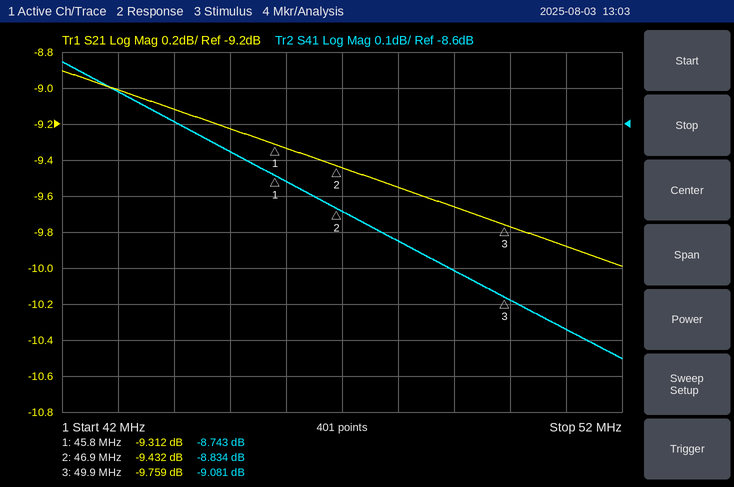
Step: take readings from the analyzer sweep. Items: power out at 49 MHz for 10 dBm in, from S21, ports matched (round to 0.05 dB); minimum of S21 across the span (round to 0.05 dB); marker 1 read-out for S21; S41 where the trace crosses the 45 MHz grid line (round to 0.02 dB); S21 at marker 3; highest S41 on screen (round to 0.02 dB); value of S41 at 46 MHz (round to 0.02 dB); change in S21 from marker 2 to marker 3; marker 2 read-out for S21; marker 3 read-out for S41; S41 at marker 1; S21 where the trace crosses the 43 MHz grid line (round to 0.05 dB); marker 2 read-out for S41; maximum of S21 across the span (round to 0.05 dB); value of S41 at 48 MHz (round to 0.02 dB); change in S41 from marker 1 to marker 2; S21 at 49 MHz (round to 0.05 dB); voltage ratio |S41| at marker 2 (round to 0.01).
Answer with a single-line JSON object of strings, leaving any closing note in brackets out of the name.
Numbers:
{"power out at 49 MHz for 10 dBm in, from S21, ports matched": "0.35 dBm", "minimum of S21 across the span": "-10.00 dB", "marker 1 read-out for S21": "-9.312 dB", "S41 where the trace crosses the 45 MHz grid line": "-8.68 dB", "S21 at marker 3": "-9.759 dB", "highest S41 on screen": "-8.42 dB", "value of S41 at 46 MHz": "-8.76 dB", "change in S21 from marker 2 to marker 3": "-0.327 dB", "marker 2 read-out for S21": "-9.432 dB", "marker 3 read-out for S41": "-9.081 dB", "S41 at marker 1": "-8.743 dB", "S21 where the trace crosses the 43 MHz grid line": "-9.00 dB", "marker 2 read-out for S41": "-8.834 dB", "maximum of S21 across the span": "-8.90 dB", "value of S41 at 48 MHz": "-8.92 dB", "change in S41 from marker 1 to marker 2": "-0.091 dB", "S21 at 49 MHz": "-9.65 dB", "voltage ratio |S41| at marker 2": "0.36"}
